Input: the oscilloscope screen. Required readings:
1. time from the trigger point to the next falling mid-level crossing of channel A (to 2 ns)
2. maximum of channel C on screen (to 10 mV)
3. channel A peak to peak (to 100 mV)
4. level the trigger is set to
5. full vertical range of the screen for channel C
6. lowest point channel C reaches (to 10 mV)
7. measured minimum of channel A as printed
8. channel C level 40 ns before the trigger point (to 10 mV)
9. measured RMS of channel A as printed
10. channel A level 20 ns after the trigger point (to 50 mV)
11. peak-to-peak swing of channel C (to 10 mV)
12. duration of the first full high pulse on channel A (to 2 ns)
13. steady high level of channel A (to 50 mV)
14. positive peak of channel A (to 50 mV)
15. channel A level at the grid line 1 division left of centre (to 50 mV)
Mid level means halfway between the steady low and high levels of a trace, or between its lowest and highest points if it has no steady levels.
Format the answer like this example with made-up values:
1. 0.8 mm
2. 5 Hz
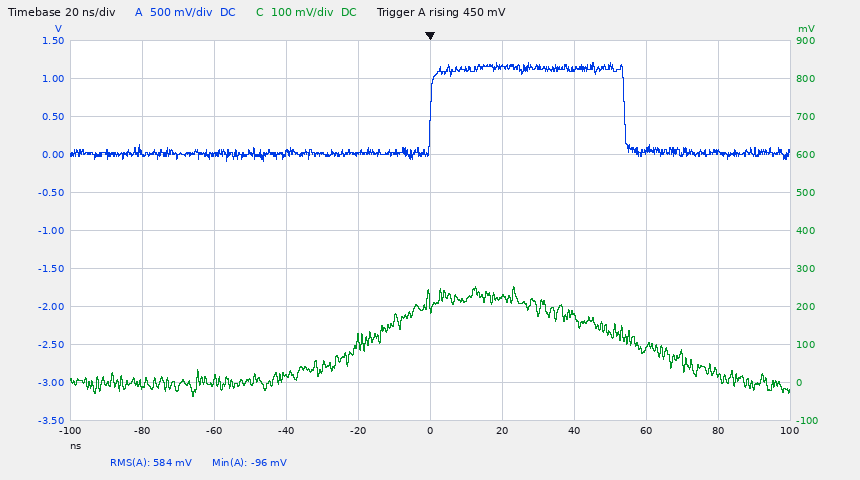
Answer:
1. 54 ns
2. 250 mV
3. 1.30 V
4. 450 mV
5. 1 V
6. -40 mV
7. -96 mV
8. 20 mV
9. 584 mV
10. 1.15 V
11. 290 mV
12. 54 ns
13. 1.15 V
14. 1.20 V
15. 0 mV
